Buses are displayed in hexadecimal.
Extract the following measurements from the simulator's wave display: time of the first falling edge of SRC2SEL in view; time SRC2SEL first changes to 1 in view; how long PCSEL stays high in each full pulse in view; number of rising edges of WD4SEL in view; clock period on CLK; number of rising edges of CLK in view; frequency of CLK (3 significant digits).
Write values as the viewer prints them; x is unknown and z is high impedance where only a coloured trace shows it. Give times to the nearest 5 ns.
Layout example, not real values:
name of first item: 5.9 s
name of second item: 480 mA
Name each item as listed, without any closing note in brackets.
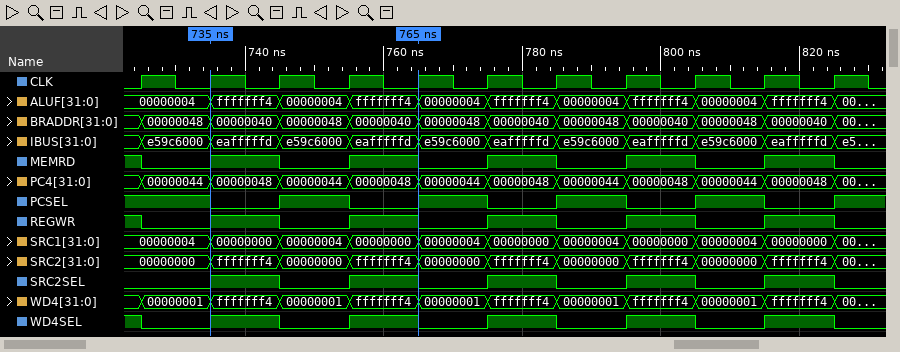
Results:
time of the first falling edge of SRC2SEL in view: 745 ns
time SRC2SEL first changes to 1 in view: 735 ns
how long PCSEL stays high in each full pulse in view: 10 ns, 10 ns, 10 ns, 10 ns
number of rising edges of WD4SEL in view: 5
clock period on CLK: 10 ns
number of rising edges of CLK in view: 11
frequency of CLK: 100 MHz
